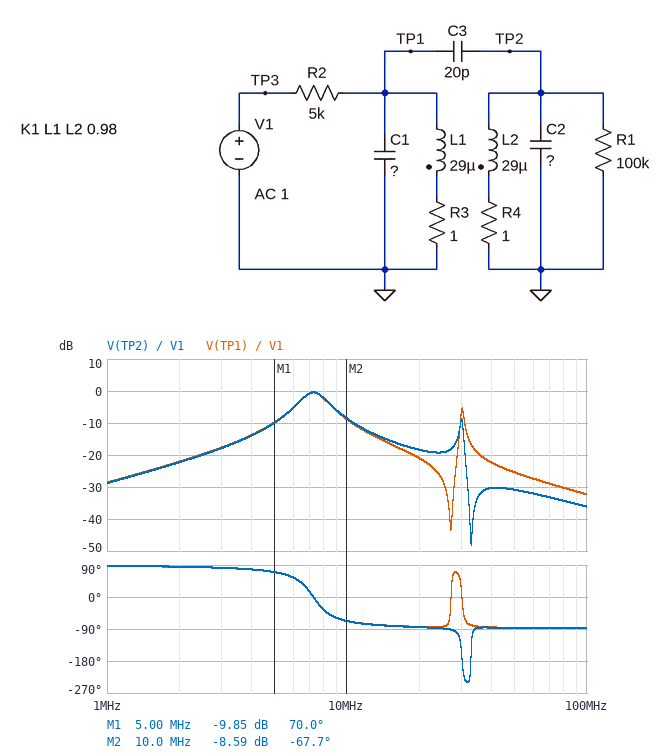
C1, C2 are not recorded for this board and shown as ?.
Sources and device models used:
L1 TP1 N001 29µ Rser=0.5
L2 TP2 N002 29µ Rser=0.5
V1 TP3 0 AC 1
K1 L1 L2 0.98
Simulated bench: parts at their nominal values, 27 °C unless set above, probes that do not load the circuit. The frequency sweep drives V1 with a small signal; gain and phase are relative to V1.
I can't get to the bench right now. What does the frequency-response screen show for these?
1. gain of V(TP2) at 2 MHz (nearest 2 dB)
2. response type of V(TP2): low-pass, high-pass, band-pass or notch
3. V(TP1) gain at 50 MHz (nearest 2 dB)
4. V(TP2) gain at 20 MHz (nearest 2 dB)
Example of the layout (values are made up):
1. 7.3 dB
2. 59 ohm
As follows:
1. -22 dB
2. band-pass
3. -26 dB
4. -18 dB
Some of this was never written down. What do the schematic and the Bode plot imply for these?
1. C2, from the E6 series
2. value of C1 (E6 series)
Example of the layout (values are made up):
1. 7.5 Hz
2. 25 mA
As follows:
1. 10 pF
2. 6.8 pF
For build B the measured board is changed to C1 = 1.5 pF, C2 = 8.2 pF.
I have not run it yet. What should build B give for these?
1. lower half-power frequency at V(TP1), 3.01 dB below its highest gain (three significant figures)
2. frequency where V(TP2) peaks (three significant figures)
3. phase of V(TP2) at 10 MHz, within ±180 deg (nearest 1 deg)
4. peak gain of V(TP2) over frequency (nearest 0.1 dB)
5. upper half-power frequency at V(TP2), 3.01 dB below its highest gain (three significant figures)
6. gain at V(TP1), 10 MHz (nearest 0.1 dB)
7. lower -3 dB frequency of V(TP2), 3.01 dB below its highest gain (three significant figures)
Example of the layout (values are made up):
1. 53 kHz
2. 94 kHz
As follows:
1. 7.96 MHz
2. 9.53 MHz
3. -16 deg
4. -0.3 dB
5. 11.4 MHz
6. -0.8 dB
7. 7.99 MHz
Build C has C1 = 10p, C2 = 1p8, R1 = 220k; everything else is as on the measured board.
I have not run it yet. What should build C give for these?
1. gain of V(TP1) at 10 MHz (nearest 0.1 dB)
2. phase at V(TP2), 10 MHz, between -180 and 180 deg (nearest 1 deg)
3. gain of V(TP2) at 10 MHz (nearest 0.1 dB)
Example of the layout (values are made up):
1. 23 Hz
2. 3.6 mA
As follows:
1. -2.9 dB
2. -43 deg
3. -3.0 dB
